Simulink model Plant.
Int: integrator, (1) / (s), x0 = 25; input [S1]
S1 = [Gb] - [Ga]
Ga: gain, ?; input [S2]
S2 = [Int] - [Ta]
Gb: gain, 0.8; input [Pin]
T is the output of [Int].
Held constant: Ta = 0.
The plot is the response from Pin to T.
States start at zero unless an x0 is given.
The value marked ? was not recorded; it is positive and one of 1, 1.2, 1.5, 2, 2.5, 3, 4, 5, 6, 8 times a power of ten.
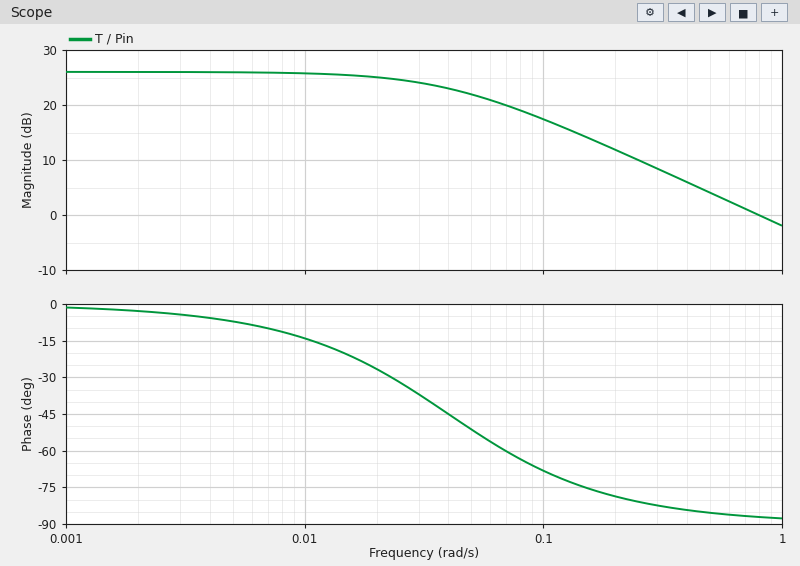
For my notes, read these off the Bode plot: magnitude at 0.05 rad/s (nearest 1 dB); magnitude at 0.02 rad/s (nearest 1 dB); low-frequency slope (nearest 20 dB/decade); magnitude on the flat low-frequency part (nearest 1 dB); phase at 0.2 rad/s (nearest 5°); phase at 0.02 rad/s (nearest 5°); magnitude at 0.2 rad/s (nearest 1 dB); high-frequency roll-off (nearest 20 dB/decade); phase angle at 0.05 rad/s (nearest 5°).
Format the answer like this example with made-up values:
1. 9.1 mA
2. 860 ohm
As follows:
1. 22 dB
2. 25 dB
3. 0 dB/decade
4. 26 dB
5. -80°
6. -25°
7. 12 dB
8. -20 dB/decade
9. -50°
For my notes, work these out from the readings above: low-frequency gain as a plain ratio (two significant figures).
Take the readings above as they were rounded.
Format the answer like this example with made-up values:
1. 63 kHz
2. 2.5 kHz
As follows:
1. 20
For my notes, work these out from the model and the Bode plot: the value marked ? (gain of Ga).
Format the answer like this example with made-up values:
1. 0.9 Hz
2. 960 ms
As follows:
1. 0.04
